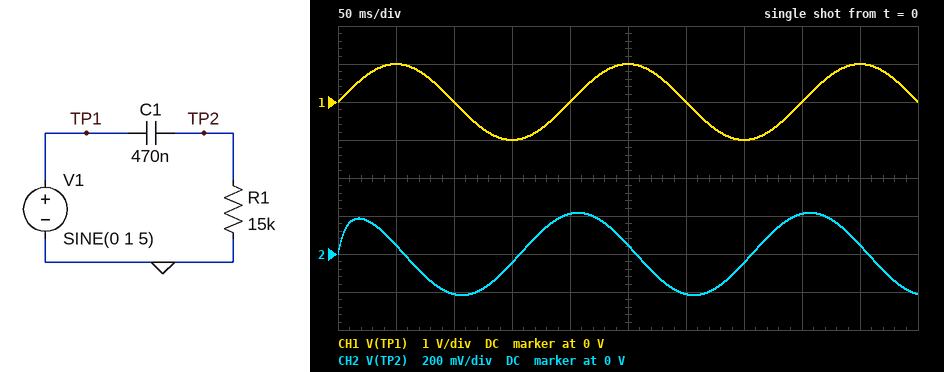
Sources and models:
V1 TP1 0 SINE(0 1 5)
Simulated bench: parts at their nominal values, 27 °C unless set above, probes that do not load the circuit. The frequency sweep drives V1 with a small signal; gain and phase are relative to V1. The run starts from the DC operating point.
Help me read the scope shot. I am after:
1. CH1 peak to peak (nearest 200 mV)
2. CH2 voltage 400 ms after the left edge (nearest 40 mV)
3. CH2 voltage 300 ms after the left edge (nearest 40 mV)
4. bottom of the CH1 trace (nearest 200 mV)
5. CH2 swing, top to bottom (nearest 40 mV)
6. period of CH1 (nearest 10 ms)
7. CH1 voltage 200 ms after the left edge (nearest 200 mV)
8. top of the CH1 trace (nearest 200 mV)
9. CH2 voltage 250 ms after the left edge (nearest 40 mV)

2.0 V
200 mV
-200 mV
-1.0 V
440 mV
200 ms
0 V
1.0 V
40 mV
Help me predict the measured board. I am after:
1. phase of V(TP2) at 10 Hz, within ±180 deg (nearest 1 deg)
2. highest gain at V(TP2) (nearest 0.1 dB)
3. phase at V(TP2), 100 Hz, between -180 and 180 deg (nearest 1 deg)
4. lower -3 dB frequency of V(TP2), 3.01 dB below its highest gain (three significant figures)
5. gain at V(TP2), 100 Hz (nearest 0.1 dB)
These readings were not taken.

66 deg
0 dB
13 deg
22.6 Hz
-0.2 dB
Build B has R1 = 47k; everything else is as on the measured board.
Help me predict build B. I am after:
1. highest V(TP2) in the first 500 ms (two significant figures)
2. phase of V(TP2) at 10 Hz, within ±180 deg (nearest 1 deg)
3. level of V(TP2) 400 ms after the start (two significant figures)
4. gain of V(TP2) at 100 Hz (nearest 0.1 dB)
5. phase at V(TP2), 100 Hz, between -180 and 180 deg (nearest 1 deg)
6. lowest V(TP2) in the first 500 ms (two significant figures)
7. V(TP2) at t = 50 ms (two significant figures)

570 mV
36 deg
470 mV
0 dB
4 deg
-570 mV
280 mV
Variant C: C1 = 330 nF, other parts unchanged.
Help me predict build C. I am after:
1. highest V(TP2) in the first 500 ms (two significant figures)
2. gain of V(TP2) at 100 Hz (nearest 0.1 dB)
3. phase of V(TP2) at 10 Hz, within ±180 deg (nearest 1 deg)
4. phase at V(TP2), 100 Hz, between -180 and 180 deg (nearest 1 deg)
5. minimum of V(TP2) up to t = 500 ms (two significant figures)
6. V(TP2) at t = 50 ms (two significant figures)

150 mV
-0.4 dB
73 deg
18 deg
-150 mV
24 mV
